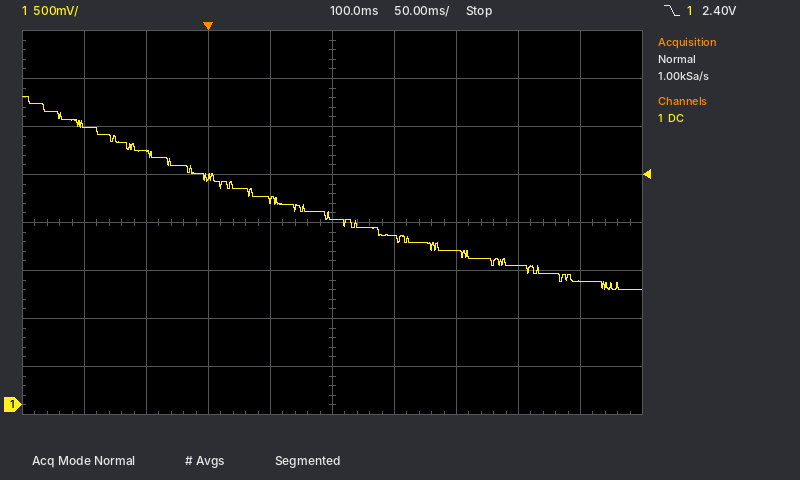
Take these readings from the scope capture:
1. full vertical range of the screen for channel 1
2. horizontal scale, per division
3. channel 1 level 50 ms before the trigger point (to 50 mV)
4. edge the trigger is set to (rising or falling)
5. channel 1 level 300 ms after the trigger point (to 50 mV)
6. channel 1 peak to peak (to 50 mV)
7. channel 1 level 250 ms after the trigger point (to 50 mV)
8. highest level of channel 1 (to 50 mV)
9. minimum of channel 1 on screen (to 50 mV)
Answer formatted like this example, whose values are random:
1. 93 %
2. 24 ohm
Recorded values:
1. 4 V
2. 50 ms
3. 2.65 V
4. falling
5. 1.30 V
6. 2.00 V
7. 1.45 V
8. 3.20 V
9. 1.20 V
